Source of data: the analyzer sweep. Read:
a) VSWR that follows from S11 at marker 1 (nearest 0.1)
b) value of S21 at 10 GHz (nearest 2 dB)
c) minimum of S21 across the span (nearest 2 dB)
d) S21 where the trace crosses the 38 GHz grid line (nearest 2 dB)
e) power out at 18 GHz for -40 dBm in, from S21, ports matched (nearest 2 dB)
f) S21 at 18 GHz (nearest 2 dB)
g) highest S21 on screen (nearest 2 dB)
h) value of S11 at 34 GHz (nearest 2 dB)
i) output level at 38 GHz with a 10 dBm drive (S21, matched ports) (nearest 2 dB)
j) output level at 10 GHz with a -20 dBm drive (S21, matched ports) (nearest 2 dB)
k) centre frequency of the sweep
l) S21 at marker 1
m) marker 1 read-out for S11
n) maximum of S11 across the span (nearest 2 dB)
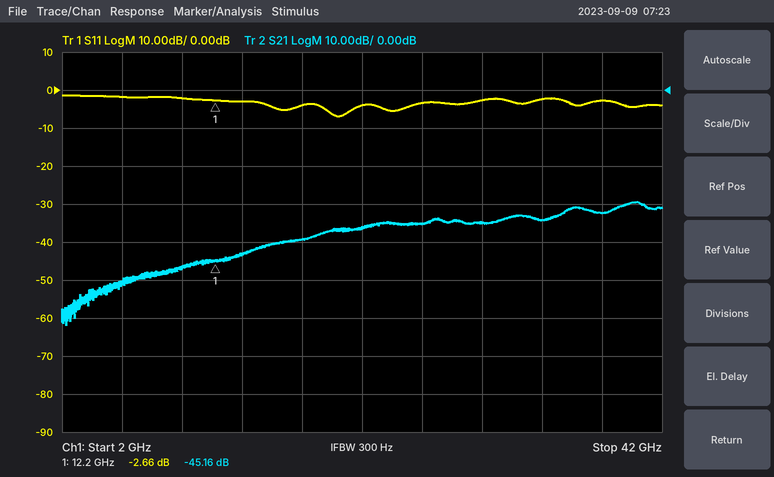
6.6
-46 dB
-62 dB
-32 dB
-80 dBm
-40 dB
-30 dB
-2 dB
-22 dBm
-66 dBm
22 GHz
-45.16 dB
-2.66 dB
-2 dB
